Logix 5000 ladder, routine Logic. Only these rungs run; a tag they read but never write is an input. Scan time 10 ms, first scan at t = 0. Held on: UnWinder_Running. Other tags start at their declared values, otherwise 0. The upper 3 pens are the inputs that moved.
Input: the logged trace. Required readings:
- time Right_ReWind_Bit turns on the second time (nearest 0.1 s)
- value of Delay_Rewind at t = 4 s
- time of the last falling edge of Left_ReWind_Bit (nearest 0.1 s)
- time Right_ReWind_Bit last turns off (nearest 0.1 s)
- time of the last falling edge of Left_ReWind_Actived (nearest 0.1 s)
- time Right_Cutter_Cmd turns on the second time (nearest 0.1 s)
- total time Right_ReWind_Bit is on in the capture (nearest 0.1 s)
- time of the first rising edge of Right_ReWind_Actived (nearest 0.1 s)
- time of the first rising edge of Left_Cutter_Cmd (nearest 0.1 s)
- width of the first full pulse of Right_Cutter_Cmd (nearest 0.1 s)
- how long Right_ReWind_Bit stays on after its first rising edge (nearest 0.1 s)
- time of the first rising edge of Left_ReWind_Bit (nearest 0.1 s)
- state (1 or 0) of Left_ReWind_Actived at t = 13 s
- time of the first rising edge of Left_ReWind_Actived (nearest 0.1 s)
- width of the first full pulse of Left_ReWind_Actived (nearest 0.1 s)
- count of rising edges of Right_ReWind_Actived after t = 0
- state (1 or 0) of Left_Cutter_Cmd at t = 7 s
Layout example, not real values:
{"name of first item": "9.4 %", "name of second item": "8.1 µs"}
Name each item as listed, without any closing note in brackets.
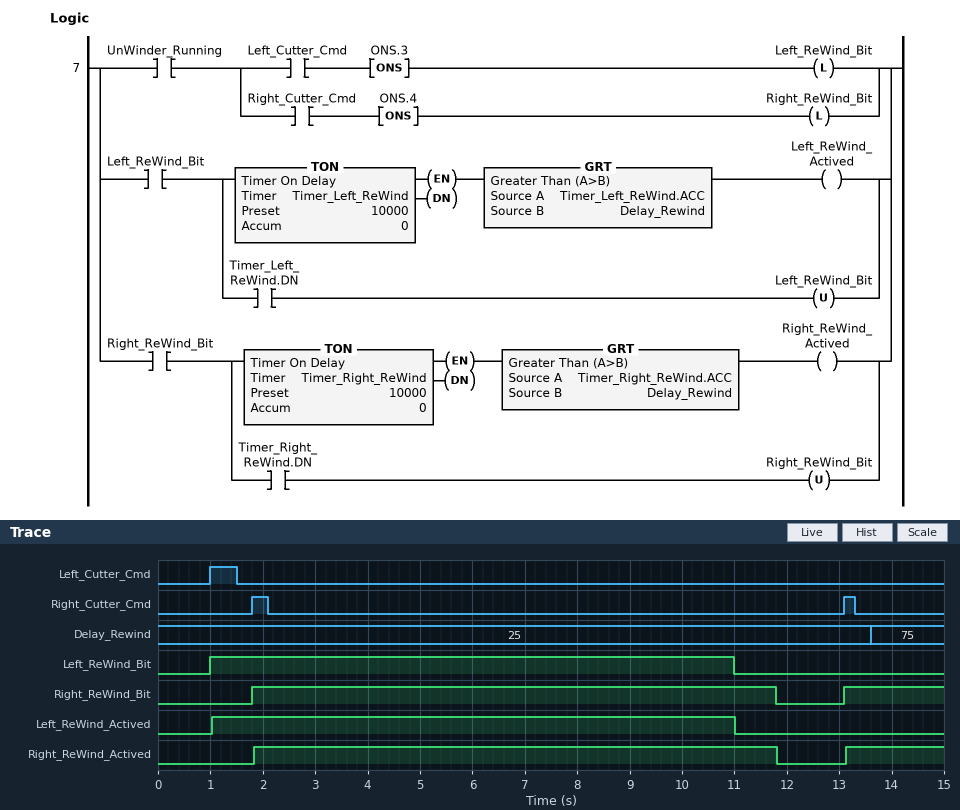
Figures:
{"time Right_ReWind_Bit turns on the second time": "13.1 s", "value of Delay_Rewind at t = 4 s": "25", "time of the last falling edge of Left_ReWind_Bit": "11.0 s", "time Right_ReWind_Bit last turns off": "11.8 s", "time of the last falling edge of Left_ReWind_Actived": "11.0 s", "time Right_Cutter_Cmd turns on the second time": "13.1 s", "total time Right_ReWind_Bit is on in the capture": "11.9 s", "time of the first rising edge of Right_ReWind_Actived": "1.8 s", "time of the first rising edge of Left_Cutter_Cmd": "1.0 s", "width of the first full pulse of Right_Cutter_Cmd": "0.3 s", "how long Right_ReWind_Bit stays on after its first rising edge": "10.0 s", "time of the first rising edge of Left_ReWind_Bit": "1.0 s", "state (1 or 0) of Left_ReWind_Actived at t = 13 s": "0", "time of the first rising edge of Left_ReWind_Actived": "1.0 s", "width of the first full pulse of Left_ReWind_Actived": "10.0 s", "count of rising edges of Right_ReWind_Actived after t = 0": "2", "state (1 or 0) of Left_Cutter_Cmd at t = 7 s": "0"}
